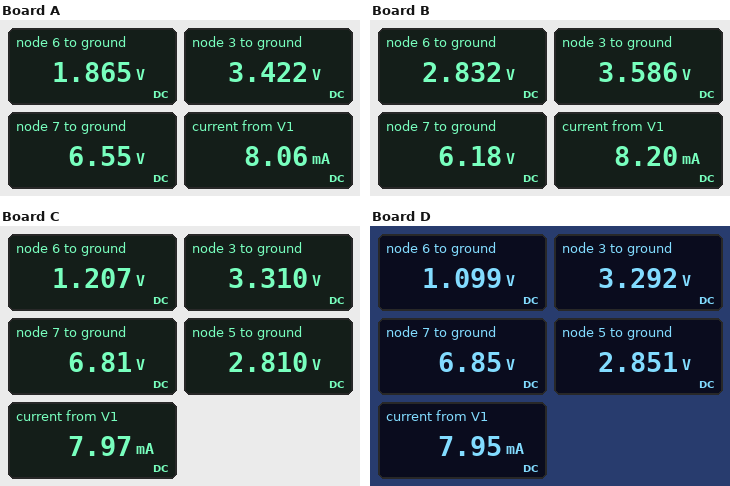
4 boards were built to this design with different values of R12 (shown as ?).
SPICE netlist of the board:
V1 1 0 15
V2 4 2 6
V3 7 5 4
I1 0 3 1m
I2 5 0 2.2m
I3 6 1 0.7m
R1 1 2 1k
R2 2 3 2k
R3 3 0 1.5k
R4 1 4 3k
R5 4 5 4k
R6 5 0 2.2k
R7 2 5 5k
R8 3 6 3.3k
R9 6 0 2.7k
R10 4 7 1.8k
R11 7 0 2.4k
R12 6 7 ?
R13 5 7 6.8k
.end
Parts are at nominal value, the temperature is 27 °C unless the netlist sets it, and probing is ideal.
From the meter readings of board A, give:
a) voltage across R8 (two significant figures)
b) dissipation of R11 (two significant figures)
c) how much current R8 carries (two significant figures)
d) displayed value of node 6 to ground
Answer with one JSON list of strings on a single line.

["1.6 V", "18 mW", "470 µA", "1.865 V"]
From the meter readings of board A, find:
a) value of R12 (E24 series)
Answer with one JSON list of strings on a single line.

["5.1 kΩ"]
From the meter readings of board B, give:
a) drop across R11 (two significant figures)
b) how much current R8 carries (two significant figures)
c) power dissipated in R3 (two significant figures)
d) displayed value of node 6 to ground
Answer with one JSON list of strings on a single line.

["6.2 V", "230 µA", "8.6 mW", "2.832 V"]
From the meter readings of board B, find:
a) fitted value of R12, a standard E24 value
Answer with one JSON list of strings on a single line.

["2.2 kΩ"]
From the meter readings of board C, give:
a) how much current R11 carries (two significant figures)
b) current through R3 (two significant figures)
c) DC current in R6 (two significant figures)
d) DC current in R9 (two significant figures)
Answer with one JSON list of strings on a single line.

["2.8 mA", "2.2 mA", "1.3 mA", "450 µA"]
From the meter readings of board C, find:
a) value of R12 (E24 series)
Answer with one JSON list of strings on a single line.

["11 kΩ"]
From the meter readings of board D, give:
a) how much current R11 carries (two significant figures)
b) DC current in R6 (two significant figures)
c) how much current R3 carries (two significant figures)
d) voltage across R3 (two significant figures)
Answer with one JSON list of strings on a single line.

["2.9 mA", "1.3 mA", "2.2 mA", "3.3 V"]
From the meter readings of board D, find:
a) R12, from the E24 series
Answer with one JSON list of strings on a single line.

["13 kΩ"]
